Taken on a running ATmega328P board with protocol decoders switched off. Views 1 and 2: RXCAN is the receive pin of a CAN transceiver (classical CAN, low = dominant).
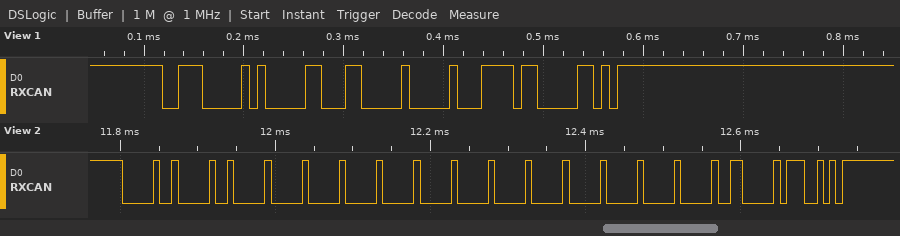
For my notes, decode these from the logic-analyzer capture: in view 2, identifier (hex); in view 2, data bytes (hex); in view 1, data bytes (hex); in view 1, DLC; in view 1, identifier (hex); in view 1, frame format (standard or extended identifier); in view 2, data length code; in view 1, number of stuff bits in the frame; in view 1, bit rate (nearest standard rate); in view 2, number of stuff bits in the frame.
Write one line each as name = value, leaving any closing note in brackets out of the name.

in view 2, identifier = 0x010
in view 2, data bytes = 00 00 00 00 00 00 00 00
in view 1, data bytes = 30 00
in view 1, DLC = 2
in view 1, identifier = 0x381
in view 1, frame format = standard
in view 2, data length code = 8
in view 1, number of stuff bits in the frame = 5
in view 1, bit rate = 125 kbit/s
in view 2, number of stuff bits in the frame = 16
